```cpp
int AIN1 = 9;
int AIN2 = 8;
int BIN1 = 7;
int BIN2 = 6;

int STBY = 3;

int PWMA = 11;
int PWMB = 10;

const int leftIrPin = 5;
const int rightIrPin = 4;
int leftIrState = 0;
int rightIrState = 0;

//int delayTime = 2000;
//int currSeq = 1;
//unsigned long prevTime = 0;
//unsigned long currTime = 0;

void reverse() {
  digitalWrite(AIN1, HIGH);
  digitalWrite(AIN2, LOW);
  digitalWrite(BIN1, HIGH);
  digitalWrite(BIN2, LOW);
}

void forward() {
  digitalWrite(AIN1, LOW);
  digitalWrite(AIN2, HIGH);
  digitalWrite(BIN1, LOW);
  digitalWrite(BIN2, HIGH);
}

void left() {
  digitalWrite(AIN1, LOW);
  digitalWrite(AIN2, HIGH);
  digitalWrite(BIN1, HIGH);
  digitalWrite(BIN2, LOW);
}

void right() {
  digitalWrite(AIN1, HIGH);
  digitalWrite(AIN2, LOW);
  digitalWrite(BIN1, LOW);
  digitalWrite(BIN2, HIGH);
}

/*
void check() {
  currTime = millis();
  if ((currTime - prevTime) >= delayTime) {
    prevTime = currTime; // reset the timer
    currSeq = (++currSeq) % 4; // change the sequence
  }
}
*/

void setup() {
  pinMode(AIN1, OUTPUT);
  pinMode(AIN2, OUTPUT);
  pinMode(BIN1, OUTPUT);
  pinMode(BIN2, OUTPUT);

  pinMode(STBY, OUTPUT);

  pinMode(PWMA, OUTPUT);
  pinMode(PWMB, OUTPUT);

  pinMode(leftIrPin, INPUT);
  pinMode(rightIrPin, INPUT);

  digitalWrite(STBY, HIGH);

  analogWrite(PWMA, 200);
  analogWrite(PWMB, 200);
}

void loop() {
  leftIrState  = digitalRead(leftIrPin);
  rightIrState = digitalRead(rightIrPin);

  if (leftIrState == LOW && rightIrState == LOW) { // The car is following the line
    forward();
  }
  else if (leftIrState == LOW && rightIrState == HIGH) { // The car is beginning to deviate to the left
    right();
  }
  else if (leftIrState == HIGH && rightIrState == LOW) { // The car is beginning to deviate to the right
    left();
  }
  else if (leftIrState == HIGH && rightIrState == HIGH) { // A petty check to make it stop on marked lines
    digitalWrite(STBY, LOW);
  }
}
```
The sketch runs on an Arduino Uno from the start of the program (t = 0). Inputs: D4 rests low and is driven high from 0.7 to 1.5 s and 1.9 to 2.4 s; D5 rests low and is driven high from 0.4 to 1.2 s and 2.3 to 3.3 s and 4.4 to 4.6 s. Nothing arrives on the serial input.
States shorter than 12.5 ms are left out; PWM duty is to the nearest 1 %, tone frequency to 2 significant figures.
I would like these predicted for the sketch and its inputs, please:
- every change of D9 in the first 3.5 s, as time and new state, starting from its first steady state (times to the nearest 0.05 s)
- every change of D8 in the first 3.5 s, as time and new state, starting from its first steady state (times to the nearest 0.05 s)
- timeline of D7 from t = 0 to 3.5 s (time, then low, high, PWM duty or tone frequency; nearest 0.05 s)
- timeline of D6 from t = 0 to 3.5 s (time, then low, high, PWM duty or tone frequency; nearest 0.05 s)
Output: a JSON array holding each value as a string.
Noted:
["0 s low; 1.2 s high; 1.5 s low; 1.9 s high; 2.4 s low", "0 s high; 1.2 s low; 1.5 s high; 1.9 s low; 2.4 s high", "0 s low; 0.4 s high; 1.2 s low; 2.4 s high; 3.3 s low", "0 s high; 0.4 s low; 1.2 s high; 2.4 s low; 3.3 s high"]
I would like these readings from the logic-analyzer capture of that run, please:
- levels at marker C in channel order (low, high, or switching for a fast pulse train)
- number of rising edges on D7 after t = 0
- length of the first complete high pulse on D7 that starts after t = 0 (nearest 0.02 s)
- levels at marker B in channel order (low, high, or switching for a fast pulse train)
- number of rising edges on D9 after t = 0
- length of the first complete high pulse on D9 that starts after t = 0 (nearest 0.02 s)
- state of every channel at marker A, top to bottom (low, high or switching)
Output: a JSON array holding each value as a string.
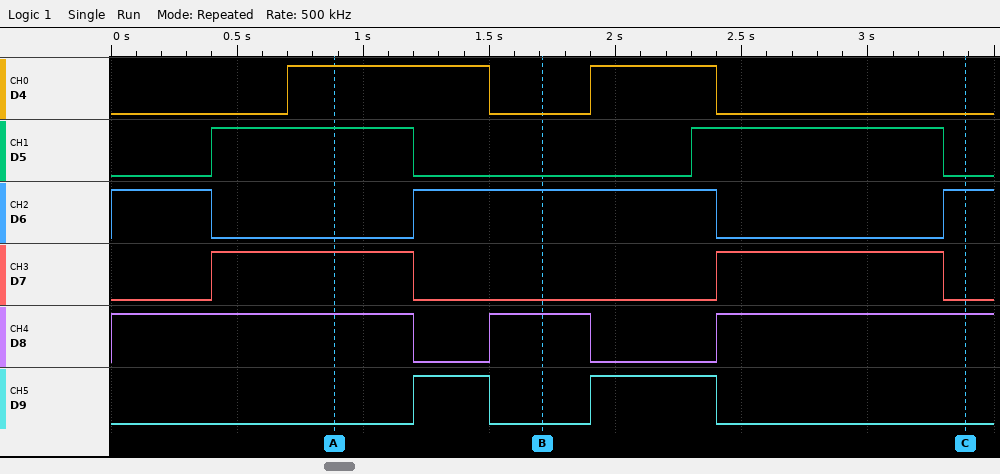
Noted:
["D4 low, D5 low, D6 high, D7 low, D8 high, D9 low", "2", "0.80 s", "D4 low, D5 low, D6 high, D7 low, D8 high, D9 low", "2", "0.30 s", "D4 high, D5 high, D6 low, D7 high, D8 high, D9 low"]
